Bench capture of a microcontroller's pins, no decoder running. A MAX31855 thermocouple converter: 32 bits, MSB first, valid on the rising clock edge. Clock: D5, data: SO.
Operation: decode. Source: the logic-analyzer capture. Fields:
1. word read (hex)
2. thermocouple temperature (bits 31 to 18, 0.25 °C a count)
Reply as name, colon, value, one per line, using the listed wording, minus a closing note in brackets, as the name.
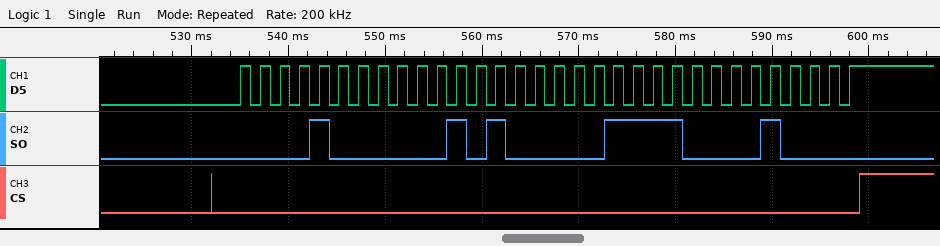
word read: 0x08141E10
thermocouple temperature: 129.25 °C
